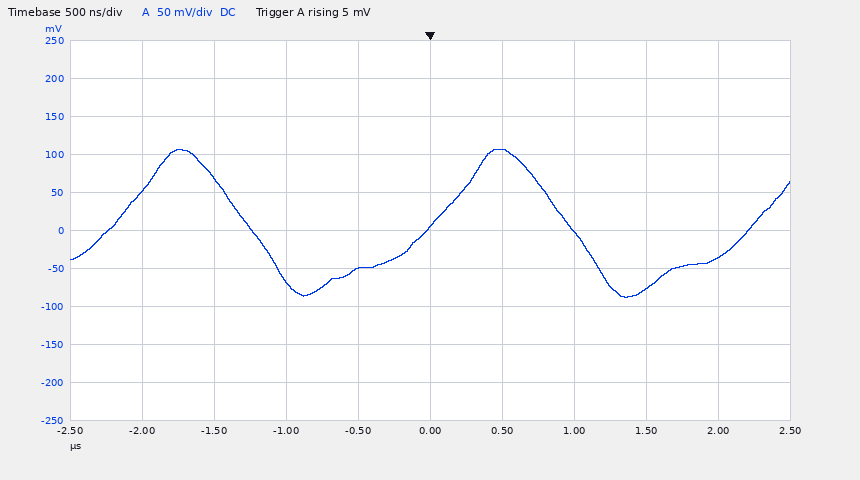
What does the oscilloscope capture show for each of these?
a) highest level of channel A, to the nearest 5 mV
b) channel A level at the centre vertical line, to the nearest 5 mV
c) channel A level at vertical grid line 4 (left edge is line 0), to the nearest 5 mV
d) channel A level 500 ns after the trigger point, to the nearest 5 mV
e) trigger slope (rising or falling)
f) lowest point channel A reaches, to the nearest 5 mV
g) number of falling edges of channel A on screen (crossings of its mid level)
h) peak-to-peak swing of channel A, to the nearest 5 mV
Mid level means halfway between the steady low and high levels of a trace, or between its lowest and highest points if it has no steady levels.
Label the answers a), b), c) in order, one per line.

a) 105 mV
b) 5 mV
c) -50 mV
d) 105 mV
e) rising
f) -90 mV
g) 2
h) 195 mV
